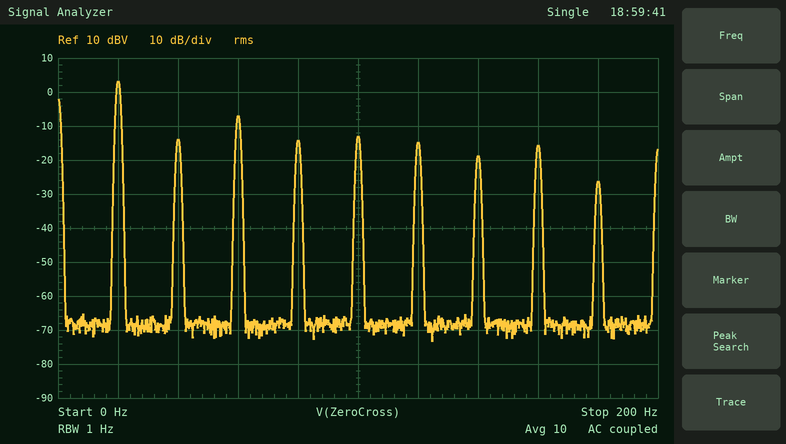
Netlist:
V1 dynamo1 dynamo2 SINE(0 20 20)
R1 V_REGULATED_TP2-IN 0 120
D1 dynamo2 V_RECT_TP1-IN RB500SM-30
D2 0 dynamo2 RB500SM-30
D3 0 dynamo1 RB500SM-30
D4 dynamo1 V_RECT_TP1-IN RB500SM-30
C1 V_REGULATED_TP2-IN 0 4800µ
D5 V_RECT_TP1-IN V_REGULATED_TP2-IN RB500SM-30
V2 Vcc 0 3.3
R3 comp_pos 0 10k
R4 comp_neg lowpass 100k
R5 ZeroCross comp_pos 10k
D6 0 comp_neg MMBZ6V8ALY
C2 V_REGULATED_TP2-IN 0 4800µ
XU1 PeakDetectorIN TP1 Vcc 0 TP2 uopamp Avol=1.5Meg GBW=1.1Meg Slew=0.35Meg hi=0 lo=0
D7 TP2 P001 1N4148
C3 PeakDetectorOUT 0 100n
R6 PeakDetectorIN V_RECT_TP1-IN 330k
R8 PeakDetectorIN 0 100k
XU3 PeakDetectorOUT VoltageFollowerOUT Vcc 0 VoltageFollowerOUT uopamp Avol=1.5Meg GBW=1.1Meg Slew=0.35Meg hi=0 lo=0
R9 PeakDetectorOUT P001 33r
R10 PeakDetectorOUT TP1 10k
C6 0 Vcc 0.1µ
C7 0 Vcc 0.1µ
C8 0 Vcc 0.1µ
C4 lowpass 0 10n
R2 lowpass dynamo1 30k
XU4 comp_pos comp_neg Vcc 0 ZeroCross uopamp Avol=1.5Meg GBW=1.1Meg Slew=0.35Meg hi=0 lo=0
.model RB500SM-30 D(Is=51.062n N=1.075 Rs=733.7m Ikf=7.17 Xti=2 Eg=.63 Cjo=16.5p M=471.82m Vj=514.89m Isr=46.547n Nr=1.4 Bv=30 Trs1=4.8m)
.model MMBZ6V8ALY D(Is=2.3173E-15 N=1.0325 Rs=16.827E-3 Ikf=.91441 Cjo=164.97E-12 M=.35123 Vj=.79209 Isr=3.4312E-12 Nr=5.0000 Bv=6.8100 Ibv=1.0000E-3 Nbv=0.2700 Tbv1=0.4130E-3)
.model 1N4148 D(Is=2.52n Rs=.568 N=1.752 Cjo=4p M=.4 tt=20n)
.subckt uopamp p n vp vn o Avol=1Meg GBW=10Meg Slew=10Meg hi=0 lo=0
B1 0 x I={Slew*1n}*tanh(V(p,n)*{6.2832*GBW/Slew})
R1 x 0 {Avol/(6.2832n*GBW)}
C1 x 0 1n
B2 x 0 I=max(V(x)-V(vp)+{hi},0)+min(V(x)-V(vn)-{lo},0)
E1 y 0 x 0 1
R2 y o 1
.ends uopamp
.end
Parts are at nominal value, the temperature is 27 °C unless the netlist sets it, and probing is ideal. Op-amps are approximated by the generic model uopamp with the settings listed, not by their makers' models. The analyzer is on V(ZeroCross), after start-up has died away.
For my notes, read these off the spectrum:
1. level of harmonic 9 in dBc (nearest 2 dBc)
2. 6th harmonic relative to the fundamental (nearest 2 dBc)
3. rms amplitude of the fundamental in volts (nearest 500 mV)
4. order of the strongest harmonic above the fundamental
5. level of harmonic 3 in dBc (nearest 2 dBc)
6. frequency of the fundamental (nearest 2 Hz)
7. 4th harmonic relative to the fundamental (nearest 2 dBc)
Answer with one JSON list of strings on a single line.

["-30 dBc", "-18 dBc", "1.5 V", "3", "-10 dBc", "20 Hz", "-18 dBc"]
